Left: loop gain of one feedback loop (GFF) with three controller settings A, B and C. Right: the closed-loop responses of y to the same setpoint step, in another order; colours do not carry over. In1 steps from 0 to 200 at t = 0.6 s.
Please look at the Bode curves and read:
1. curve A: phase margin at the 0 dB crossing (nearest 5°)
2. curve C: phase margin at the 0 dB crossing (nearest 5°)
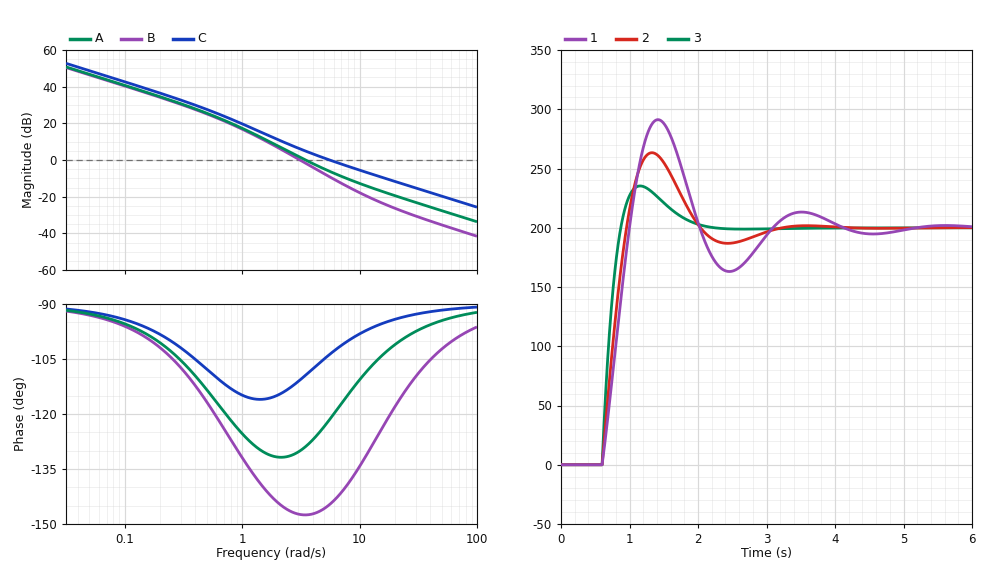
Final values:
50°
75°
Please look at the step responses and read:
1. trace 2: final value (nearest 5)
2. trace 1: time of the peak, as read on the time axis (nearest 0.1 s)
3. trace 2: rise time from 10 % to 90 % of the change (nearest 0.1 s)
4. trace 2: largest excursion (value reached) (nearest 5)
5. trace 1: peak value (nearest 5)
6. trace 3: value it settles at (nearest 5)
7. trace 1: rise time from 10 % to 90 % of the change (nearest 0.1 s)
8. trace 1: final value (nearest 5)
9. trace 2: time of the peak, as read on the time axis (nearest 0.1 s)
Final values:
200
1.4 s
0.3 s
265
290
200
0.3 s
200
1.3 s
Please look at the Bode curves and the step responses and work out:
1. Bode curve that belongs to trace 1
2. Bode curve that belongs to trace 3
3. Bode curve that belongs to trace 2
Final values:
B
C
A
